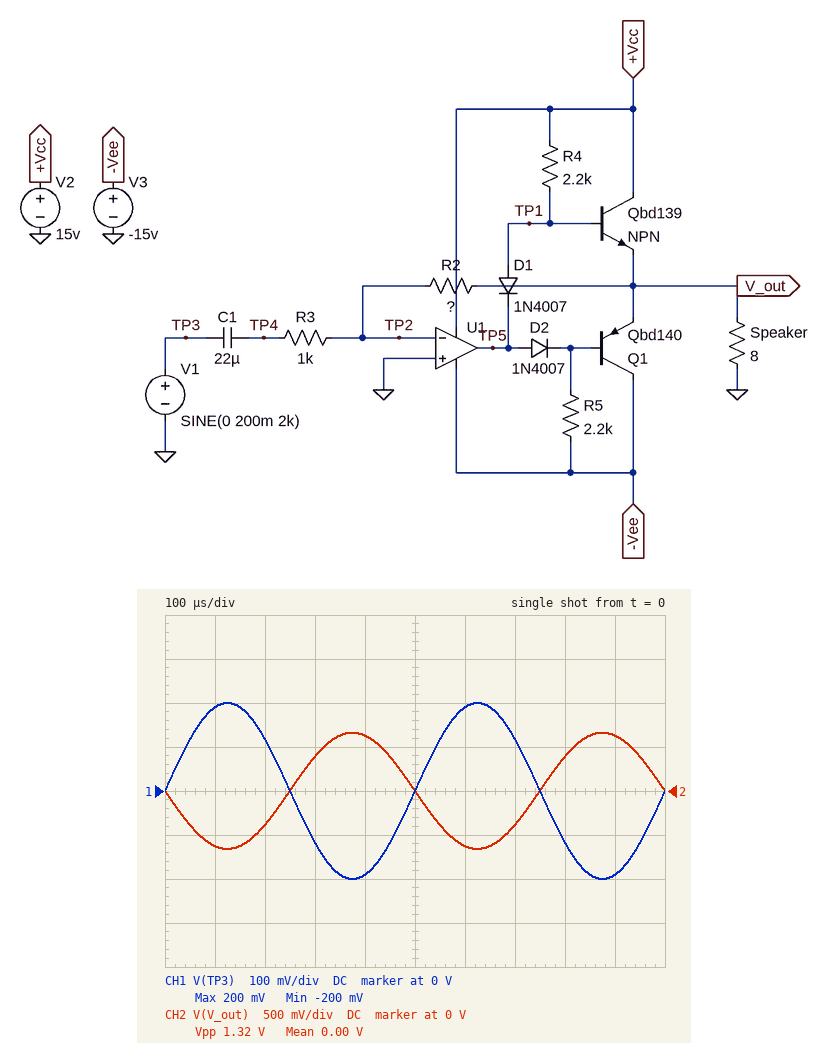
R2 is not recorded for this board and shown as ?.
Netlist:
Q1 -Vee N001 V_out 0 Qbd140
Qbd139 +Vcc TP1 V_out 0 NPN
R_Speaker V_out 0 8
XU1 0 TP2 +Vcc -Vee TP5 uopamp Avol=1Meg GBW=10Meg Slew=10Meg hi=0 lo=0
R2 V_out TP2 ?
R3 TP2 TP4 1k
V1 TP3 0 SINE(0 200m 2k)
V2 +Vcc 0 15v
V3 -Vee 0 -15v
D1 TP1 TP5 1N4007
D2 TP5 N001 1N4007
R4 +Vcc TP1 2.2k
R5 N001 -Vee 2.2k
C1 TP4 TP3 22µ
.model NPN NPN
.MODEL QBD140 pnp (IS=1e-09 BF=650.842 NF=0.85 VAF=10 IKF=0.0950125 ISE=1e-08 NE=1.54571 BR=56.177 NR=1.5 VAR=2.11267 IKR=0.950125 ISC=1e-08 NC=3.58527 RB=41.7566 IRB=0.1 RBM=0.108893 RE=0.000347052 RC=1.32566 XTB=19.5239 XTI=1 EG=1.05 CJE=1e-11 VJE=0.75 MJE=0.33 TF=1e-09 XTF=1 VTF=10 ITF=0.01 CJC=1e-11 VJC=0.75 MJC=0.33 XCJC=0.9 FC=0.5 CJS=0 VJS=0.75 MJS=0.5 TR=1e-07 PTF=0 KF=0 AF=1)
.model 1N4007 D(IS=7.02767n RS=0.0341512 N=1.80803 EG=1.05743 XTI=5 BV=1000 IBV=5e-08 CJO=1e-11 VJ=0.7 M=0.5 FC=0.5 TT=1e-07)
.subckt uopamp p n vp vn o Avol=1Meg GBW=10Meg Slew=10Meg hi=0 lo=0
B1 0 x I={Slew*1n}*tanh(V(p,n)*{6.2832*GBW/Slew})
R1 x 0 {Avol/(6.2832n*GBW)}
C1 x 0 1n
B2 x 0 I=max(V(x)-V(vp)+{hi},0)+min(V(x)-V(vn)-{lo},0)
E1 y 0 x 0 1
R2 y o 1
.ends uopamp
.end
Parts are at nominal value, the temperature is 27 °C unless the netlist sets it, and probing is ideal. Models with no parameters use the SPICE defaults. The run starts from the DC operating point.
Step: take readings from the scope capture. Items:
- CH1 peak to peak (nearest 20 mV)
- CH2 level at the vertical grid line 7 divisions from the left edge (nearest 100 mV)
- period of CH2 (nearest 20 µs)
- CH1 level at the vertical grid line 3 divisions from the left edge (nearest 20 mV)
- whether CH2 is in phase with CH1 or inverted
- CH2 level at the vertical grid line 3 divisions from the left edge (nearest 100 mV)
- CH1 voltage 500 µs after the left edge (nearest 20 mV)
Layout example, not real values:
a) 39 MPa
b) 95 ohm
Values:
a) 400 mV
b) -400 mV
c) 500 µs
d) -120 mV
e) inverted
f) 400 mV
g) 0 V
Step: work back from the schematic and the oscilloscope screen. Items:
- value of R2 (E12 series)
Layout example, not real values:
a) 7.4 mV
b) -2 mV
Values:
a) 3.3 kΩ
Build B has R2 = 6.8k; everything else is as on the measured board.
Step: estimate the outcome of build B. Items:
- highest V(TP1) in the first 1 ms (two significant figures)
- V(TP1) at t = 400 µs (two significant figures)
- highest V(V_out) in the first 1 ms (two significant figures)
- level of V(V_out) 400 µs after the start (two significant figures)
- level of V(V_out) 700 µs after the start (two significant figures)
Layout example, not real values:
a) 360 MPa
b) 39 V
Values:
a) 2.3 V
b) 2.2 V
c) 1.4 V
d) 1.3 V
e) -790 mV
